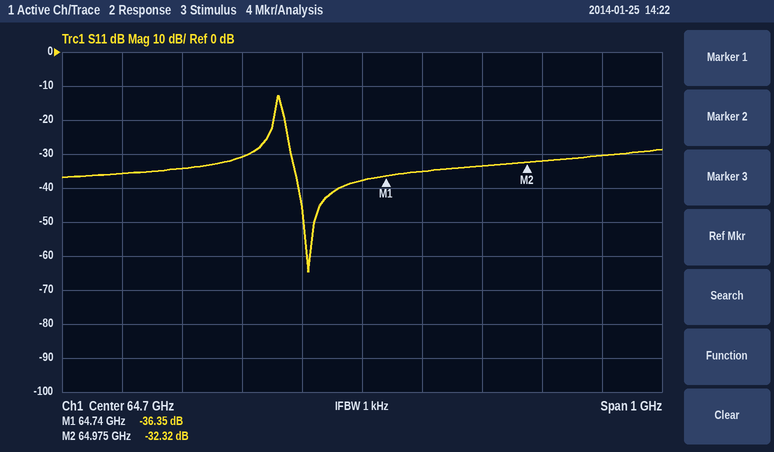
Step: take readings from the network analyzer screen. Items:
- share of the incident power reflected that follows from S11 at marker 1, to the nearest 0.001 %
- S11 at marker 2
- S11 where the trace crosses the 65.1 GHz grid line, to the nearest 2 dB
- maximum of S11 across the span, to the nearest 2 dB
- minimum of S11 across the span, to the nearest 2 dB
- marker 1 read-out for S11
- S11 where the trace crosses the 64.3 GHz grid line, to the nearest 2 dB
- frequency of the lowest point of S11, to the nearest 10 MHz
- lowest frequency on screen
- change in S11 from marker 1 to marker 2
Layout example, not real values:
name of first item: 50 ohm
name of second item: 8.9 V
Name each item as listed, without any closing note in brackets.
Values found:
share of the incident power reflected that follows from S11 at marker 1, to the nearest 0.001 %: 0.023 %
S11 at marker 2: -32.32 dB
S11 where the trace crosses the 65.1 GHz grid line, to the nearest 2 dB: -30 dB
maximum of S11 across the span, to the nearest 2 dB: -12 dB
minimum of S11 across the span, to the nearest 2 dB: -64 dB
marker 1 read-out for S11: -36.35 dB
S11 where the trace crosses the 64.3 GHz grid line, to the nearest 2 dB: -36 dB
frequency of the lowest point of S11, to the nearest 10 MHz: 64.61 GHz
lowest frequency on screen: 64.2 GHz
change in S11 from marker 1 to marker 2: 4.03 dB
